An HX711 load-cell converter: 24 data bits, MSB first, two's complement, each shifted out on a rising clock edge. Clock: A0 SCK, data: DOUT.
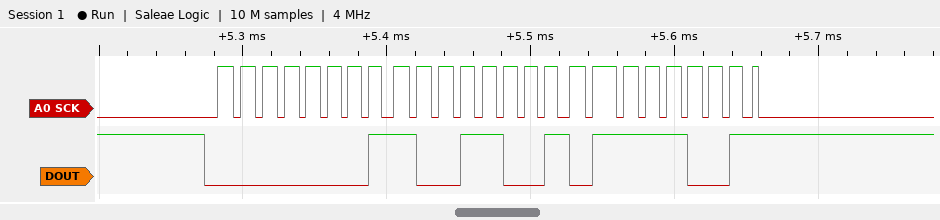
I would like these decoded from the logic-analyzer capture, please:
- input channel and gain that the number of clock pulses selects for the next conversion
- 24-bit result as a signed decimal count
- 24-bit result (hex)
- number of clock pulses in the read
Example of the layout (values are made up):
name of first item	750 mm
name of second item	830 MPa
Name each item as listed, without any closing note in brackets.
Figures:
input channel and gain that the number of clock pulses selects for the next conversion	channel A, gain 128
24-bit result as a signed decimal count	104825
24-bit result	0x019979
number of clock pulses in the read	25
